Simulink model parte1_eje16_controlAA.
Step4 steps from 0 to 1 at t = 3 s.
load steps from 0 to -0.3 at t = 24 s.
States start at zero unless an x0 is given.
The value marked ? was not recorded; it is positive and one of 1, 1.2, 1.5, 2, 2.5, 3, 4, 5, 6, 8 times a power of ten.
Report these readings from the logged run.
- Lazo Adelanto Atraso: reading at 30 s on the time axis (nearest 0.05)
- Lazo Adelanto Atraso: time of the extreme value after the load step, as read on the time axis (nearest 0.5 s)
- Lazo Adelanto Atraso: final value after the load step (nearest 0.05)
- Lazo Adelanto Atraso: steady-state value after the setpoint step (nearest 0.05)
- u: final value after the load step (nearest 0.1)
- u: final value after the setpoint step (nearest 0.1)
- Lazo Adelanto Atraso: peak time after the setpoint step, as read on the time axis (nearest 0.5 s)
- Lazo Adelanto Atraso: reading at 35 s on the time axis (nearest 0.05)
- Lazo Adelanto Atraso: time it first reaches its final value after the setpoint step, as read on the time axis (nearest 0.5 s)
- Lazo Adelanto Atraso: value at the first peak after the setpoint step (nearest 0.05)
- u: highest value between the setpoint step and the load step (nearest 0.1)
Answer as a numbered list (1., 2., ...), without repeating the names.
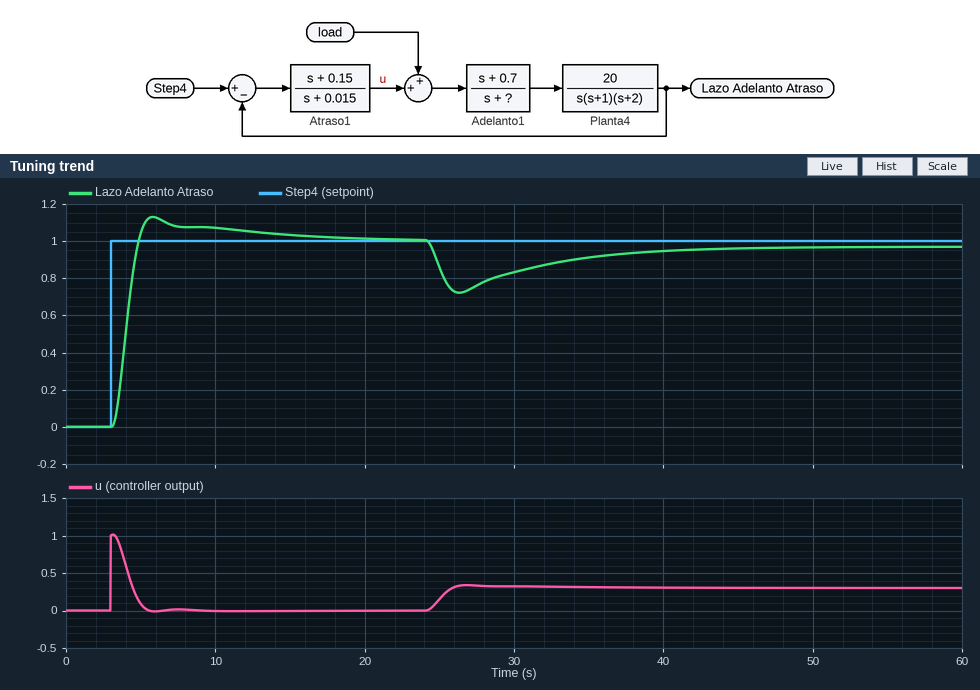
1. 0.85
2. 26.5 s
3. 0.95
4. 1.00
5. 0.3
6. 0.0
7. 6.0 s
8. 0.90
9. 5.0 s
10. 1.15
11. 1.0
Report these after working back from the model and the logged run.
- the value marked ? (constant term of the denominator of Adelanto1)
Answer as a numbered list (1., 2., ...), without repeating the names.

1. 8
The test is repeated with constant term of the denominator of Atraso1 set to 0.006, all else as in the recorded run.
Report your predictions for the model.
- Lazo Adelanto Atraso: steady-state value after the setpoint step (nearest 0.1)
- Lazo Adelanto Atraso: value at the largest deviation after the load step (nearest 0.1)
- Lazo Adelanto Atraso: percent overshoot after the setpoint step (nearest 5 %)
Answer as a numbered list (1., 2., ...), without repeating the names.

1. 1.0
2. 0.7
3. 15 %
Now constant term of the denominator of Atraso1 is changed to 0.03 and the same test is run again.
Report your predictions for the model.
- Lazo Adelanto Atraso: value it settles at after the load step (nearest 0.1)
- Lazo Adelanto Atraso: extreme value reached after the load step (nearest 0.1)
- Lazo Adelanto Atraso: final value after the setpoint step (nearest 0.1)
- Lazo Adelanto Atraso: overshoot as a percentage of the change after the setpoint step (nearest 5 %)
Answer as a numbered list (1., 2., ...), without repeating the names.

1. 0.9
2. 0.7
3. 1.0
4. 10 %
